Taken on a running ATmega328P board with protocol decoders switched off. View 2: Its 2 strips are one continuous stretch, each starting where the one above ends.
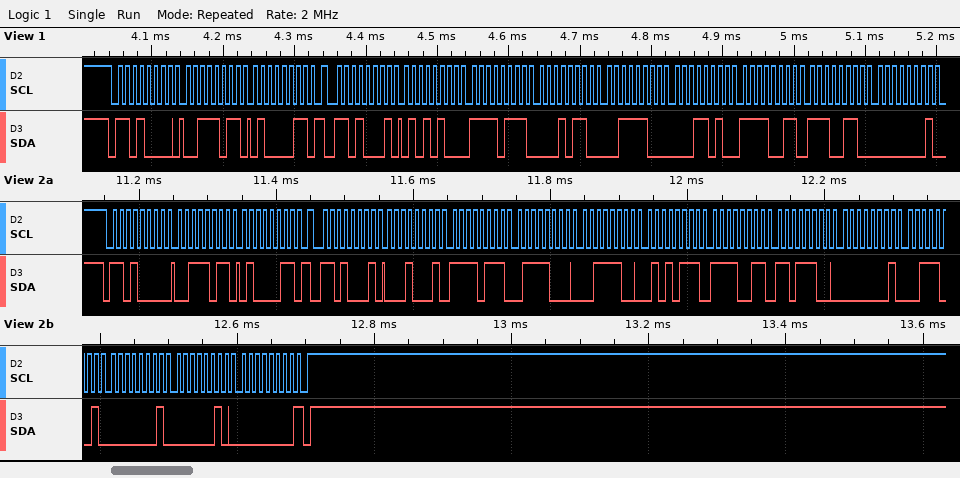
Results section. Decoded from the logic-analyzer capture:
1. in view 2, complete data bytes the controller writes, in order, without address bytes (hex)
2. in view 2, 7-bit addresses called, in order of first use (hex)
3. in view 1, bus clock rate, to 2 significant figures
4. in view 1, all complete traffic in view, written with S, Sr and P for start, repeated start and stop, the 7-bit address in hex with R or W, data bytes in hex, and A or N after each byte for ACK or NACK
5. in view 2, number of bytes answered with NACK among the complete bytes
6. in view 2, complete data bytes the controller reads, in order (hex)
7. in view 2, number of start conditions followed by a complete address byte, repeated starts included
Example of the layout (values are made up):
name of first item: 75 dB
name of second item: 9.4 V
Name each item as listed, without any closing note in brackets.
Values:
in view 2, complete data bytes the controller writes, in order, without address bytes: 3B 43
in view 2, 7-bit addresses called, in order of first use: 0x68
in view 1, bus clock rate, to 2 significant figures: 100 kHz
in view 1, all complete traffic in view, written with S, Sr and P for start, repeated start and stop, the 7-bit address in hex with R or W, data bytes in hex, and A or N after each byte for ACK or NACK: S 68W A 3B A 43 A Sr 68R A 54 A F7 A 16 A 3C A 1A A F3 A E6 A 01 A
in view 2, number of bytes answered with NACK among the complete bytes: 1
in view 2, complete data bytes the controller reads, in order: 11 F7 78 3C 57 F3 DC 01 39 01 02 00
in view 2, number of start conditions followed by a complete address byte, repeated starts included: 2
